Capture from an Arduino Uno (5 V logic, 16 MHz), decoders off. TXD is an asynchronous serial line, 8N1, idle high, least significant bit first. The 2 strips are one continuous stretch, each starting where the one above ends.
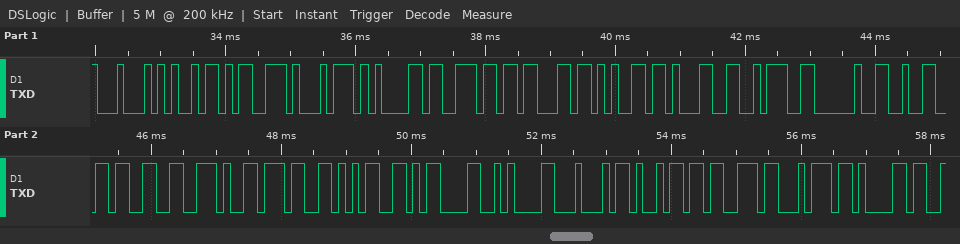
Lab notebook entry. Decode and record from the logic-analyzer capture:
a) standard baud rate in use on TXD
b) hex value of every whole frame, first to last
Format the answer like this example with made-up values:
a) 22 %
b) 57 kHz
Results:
a) 9600 baud
b) 44 69 73 74 61 6E 63 65 31 3A 20 32 33 2E 37 35 0D 0A 44 69 73 74 61
